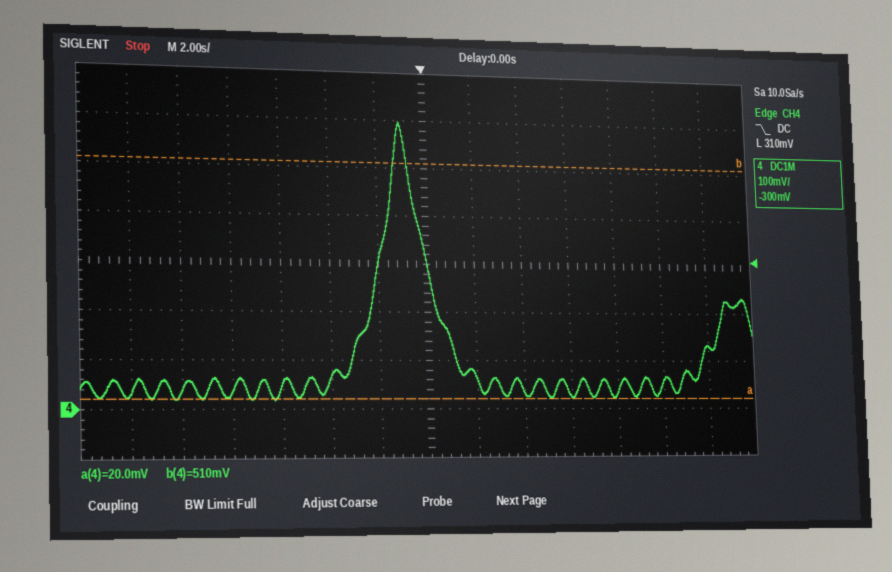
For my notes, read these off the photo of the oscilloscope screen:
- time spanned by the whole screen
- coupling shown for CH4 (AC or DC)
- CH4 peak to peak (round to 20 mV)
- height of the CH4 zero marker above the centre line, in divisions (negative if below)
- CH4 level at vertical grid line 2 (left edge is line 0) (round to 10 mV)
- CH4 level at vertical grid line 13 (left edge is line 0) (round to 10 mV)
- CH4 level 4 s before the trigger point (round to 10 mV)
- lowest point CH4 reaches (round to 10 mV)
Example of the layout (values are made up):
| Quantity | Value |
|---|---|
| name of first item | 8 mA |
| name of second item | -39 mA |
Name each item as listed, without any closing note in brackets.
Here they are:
| Quantity | Value |
|---|---|
| time spanned by the whole screen | 28 s |
| coupling shown for CH4 | DC |
| CH4 peak to peak | 580 mV |
| height of the CH4 zero marker above the centre line, in divisions | -3.0 div |
| CH4 level at vertical grid line 2 (left edge is line 0) | 40 mV |
| CH4 level at vertical grid line 13 (left edge is line 0) | 130 mV |
| CH4 level 4 s before the trigger point | 70 mV |
| lowest point CH4 reaches | 20 mV |
